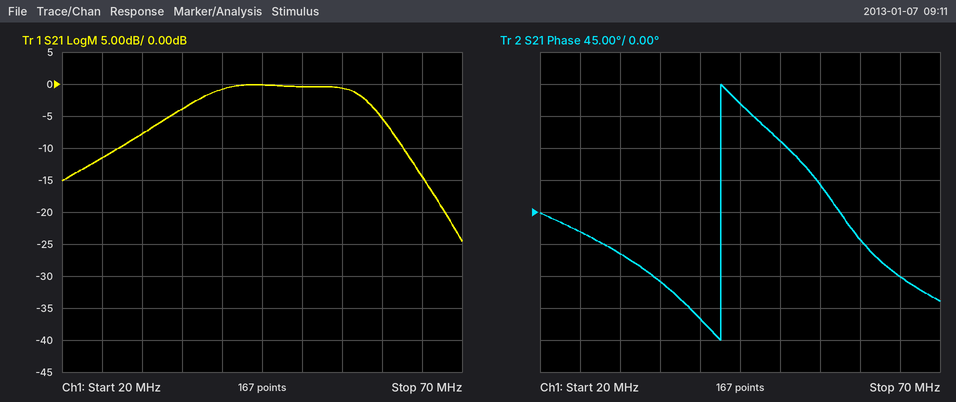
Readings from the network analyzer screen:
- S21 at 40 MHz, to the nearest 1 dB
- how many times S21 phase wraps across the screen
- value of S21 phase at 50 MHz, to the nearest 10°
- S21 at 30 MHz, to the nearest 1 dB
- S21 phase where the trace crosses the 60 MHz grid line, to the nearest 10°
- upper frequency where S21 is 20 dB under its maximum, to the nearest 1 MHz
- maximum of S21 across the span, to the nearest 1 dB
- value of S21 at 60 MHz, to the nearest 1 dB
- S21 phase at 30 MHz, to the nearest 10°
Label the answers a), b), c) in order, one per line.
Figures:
a) -1 dB
b) 1
c) 100°
d) -8 dB
e) -40°
f) 68 MHz
g) 0 dB
h) -5 dB
i) -60°
